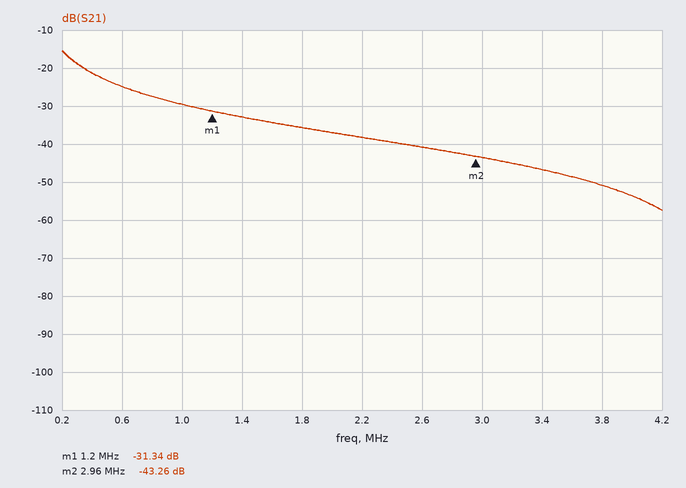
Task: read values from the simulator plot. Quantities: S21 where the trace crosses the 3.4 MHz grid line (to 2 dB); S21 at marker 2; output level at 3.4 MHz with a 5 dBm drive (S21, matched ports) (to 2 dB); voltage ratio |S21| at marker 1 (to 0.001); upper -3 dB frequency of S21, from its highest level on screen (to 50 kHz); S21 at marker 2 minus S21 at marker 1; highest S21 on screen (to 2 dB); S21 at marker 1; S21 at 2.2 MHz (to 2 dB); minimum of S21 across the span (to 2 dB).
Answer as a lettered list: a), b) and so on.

a) -46 dB
b) -43.26 dB
c) -42 dBm
d) 0.027
e) 300 kHz
f) -11.92 dB
g) -16 dB
h) -31.34 dB
i) -38 dB
j) -58 dB
